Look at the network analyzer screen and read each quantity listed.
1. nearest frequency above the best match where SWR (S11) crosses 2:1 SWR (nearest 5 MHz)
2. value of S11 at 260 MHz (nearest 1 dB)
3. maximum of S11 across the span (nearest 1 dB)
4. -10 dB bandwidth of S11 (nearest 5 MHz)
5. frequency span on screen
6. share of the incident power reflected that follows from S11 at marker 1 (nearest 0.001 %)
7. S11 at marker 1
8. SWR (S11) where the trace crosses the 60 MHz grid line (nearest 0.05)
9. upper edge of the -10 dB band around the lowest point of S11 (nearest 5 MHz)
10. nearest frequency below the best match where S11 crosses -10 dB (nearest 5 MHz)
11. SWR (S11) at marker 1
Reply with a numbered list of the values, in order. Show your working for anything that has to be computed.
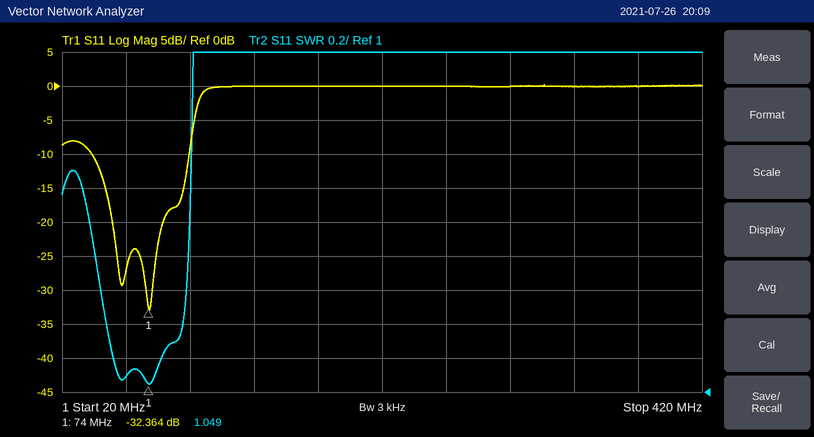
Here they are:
1. 100 MHz
2. 0 dB
3. 0 dB
4. 100 MHz − 40 MHz = 60 MHz
5. 400 MHz
6. 10^(-32.364/10) ≈ 0.058 %
7. -32.364 dB
8. 1.10
9. 100 MHz
10. 40 MHz
11. 1.049
